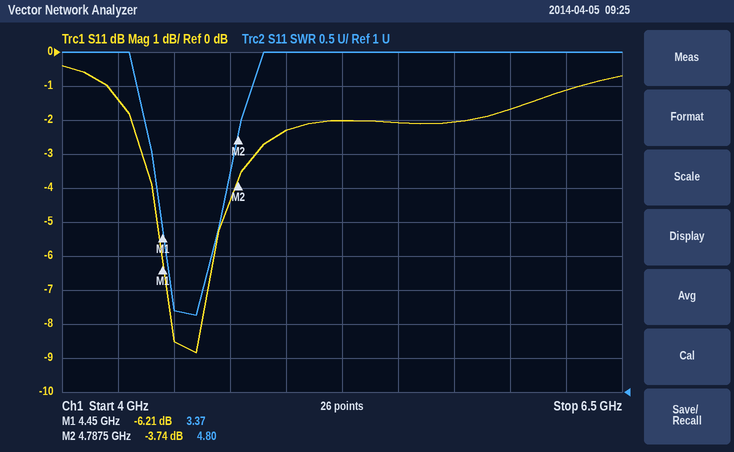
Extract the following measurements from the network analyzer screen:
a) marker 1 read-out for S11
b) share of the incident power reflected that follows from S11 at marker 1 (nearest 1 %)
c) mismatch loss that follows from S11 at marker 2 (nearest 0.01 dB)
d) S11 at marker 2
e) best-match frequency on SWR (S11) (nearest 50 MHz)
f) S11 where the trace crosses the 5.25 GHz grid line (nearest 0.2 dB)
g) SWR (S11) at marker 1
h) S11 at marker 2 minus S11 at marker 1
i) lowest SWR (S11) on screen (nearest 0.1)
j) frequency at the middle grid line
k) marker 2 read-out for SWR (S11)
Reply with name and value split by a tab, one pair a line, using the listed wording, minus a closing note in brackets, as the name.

marker 1 read-out for S11	-6.21 dB
share of the incident power reflected that follows from S11 at marker 1	24 %
mismatch loss that follows from S11 at marker 2	2.39 dB
S11 at marker 2	-3.74 dB
best-match frequency on SWR (S11)	4.60 GHz
S11 where the trace crosses the 5.25 GHz grid line	-2.0 dB
SWR (S11) at marker 1	3.37
S11 at marker 2 minus S11 at marker 1	2.47 dB
lowest SWR (S11) on screen	2.1
frequency at the middle grid line	5.25 GHz
marker 2 read-out for SWR	4.80
